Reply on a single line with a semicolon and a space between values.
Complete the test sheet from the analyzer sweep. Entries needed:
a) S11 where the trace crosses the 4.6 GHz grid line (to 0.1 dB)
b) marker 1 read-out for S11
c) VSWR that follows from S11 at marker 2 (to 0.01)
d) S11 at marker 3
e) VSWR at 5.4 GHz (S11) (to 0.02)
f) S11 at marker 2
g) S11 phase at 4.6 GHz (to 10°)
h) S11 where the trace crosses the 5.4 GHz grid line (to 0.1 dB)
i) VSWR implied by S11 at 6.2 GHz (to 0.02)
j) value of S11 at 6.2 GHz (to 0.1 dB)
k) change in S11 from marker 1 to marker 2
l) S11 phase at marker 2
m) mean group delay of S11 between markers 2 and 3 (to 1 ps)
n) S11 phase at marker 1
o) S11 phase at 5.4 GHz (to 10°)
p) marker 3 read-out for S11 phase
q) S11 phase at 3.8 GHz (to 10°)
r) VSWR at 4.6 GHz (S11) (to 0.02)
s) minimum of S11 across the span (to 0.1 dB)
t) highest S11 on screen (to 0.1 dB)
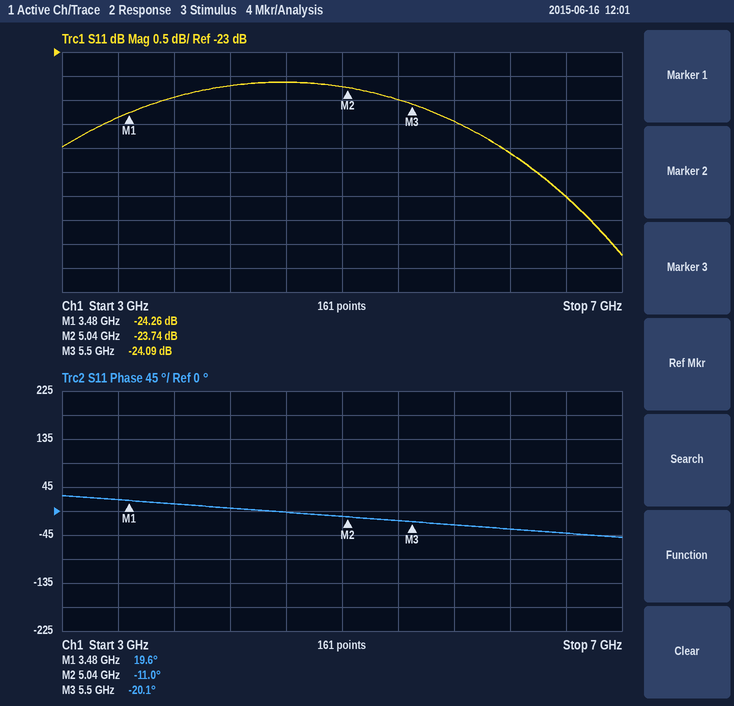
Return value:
-23.6 dB; -24.26 dB; 1.14; -24.09 dB; 1.14; -23.74 dB; 0°; -24.0 dB; 1.12; -25.1 dB; 0.52 dB; -11.0°; 55 ps; 19.6°; -20°; -20.1°; 10°; 1.14; -27.2 dB; -23.6 dB
